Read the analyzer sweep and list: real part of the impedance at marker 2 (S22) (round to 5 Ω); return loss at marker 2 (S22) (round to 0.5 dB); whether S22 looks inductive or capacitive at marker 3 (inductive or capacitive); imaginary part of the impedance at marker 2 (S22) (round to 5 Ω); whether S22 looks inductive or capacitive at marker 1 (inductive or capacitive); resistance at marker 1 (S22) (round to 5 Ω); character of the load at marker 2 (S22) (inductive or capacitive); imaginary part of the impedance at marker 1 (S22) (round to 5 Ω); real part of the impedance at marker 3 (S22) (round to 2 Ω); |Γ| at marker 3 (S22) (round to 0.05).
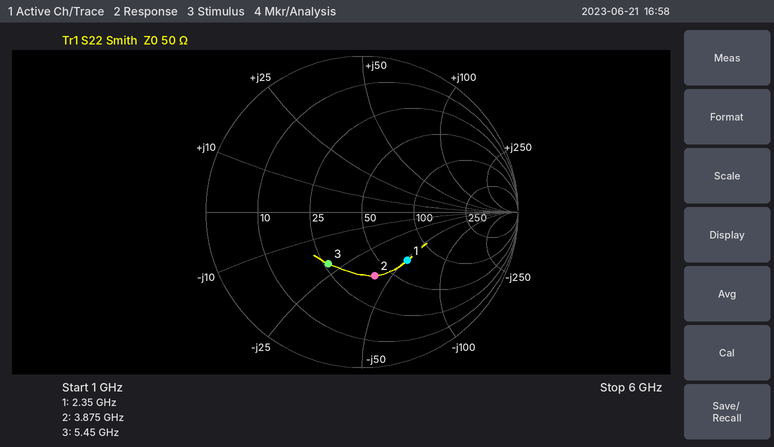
40 Ω
7.5 dB
capacitive
-40 Ω
capacitive
70 Ω
capacitive
-50 Ω
26 Ω
0.40
